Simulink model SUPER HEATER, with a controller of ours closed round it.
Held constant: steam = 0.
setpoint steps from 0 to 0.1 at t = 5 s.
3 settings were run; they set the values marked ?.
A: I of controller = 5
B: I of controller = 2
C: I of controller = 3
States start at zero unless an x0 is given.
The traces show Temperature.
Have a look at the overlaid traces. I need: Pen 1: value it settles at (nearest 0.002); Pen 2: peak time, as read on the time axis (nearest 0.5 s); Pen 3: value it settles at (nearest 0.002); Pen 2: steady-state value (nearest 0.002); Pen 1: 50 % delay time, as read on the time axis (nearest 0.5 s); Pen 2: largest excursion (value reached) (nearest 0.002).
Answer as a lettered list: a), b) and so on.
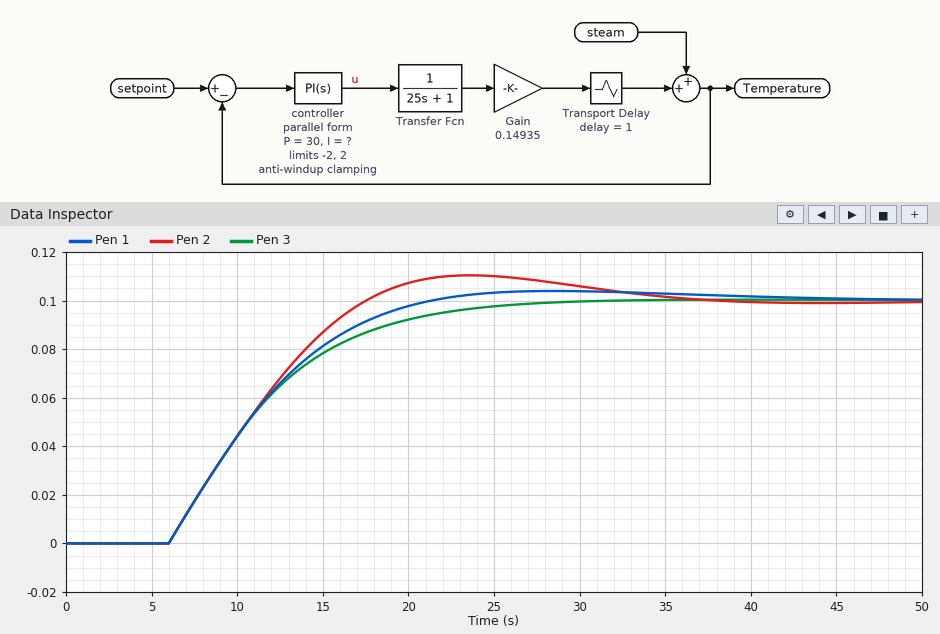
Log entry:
a) 0.100
b) 23.5 s
c) 0.100
d) 0.100
e) 10.5 s
f) 0.110
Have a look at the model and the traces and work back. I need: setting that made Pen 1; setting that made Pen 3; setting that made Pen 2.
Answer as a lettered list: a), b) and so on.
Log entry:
a) C
b) B
c) A
